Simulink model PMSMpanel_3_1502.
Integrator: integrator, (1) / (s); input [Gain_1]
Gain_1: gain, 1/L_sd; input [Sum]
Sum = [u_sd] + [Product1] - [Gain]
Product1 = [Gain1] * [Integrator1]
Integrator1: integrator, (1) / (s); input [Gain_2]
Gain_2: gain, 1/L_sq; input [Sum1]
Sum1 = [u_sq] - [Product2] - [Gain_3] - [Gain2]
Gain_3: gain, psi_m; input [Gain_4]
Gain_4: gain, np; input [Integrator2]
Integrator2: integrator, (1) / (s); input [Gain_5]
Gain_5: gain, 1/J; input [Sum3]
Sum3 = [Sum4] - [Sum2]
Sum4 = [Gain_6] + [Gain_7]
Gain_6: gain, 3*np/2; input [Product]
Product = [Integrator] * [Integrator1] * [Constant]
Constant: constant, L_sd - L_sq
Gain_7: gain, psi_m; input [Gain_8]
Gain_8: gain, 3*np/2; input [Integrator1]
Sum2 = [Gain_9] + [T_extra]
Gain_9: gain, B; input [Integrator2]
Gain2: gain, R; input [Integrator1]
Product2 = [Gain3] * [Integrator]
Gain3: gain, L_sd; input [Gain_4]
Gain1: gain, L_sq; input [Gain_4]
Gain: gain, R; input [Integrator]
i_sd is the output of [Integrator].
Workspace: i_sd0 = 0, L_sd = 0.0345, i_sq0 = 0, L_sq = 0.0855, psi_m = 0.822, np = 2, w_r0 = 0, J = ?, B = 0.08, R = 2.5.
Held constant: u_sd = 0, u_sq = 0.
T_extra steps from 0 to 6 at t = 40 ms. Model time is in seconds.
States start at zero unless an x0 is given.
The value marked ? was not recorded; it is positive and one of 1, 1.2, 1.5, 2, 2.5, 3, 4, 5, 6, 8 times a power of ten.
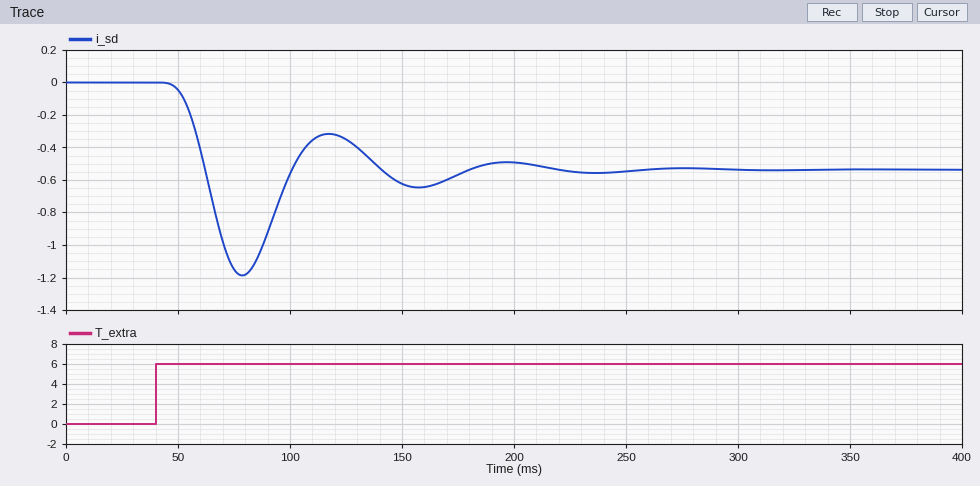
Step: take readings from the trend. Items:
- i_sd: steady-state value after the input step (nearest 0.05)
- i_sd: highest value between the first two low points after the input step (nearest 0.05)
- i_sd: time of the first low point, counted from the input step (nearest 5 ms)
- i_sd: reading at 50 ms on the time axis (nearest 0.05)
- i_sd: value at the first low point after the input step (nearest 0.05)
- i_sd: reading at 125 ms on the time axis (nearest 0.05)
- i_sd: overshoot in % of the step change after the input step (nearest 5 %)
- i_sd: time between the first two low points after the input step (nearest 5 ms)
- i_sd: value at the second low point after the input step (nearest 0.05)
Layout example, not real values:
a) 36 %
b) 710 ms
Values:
a) -0.55
b) -0.30
c) 40 ms
d) -0.05
e) -1.20
f) -0.35
g) 120 %
h) 80 ms
i) -0.65
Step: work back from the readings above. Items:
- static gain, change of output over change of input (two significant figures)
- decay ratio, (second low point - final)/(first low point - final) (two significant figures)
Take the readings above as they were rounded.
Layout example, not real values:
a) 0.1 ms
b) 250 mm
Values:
a) -0.092
b) 0.15
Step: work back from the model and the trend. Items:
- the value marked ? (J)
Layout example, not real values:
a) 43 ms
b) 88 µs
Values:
a) 0.008
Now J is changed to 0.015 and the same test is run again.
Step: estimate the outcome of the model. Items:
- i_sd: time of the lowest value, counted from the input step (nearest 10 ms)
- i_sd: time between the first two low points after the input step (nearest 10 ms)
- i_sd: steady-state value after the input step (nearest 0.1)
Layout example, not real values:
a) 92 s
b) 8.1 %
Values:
a) 50 ms
b) 110 ms
c) -0.5
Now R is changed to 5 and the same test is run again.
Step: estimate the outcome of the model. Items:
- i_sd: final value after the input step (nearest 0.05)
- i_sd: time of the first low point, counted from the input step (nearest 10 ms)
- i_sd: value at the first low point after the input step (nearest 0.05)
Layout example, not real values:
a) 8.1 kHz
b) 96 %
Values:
a) -0.50
b) 40 ms
c) -0.75
